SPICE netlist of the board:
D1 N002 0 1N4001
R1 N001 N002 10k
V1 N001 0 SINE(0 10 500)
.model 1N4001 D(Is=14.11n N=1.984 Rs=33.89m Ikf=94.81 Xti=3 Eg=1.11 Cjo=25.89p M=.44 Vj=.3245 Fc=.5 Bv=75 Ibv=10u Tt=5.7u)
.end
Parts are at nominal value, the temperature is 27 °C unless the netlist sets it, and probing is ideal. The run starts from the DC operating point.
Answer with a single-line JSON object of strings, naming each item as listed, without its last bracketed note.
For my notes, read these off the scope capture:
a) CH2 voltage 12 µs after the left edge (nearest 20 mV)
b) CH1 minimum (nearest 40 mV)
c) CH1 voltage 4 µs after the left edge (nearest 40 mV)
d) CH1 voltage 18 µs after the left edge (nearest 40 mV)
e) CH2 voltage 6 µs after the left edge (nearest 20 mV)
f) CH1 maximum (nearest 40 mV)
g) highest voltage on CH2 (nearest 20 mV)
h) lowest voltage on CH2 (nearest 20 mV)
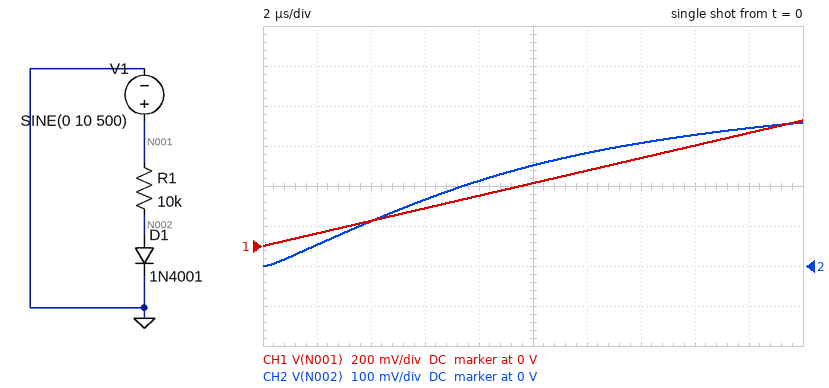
{"CH2 voltage 12 µs after the left edge": "280 mV", "CH1 minimum": "0 V", "CH1 voltage 4 µs after the left edge": "120 mV", "CH1 voltage 18 µs after the left edge": "560 mV", "CH2 voltage 6 µs after the left edge": "160 mV", "CH1 maximum": "640 mV", "highest voltage on CH2": "360 mV", "lowest voltage on CH2": "0 V"}
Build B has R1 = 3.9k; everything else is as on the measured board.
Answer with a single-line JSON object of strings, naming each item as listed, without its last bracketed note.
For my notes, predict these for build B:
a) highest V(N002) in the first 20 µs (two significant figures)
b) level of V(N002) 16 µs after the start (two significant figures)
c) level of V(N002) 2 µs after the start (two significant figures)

{"highest V(N002) in the first 20 µs": "400 mV", "level of V(N002) 16 µs after the start": "360 mV", "level of V(N002) 2 µs after the start": "59 mV"}
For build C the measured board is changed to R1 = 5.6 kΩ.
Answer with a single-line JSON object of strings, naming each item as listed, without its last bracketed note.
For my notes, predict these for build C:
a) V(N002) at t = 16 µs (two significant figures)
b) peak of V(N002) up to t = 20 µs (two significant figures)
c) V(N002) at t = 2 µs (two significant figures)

{"V(N002) at t = 16 µs": "350 mV", "peak of V(N002) up to t = 20 µs": "380 mV", "V(N002) at t = 2 µs": "57 mV"}
